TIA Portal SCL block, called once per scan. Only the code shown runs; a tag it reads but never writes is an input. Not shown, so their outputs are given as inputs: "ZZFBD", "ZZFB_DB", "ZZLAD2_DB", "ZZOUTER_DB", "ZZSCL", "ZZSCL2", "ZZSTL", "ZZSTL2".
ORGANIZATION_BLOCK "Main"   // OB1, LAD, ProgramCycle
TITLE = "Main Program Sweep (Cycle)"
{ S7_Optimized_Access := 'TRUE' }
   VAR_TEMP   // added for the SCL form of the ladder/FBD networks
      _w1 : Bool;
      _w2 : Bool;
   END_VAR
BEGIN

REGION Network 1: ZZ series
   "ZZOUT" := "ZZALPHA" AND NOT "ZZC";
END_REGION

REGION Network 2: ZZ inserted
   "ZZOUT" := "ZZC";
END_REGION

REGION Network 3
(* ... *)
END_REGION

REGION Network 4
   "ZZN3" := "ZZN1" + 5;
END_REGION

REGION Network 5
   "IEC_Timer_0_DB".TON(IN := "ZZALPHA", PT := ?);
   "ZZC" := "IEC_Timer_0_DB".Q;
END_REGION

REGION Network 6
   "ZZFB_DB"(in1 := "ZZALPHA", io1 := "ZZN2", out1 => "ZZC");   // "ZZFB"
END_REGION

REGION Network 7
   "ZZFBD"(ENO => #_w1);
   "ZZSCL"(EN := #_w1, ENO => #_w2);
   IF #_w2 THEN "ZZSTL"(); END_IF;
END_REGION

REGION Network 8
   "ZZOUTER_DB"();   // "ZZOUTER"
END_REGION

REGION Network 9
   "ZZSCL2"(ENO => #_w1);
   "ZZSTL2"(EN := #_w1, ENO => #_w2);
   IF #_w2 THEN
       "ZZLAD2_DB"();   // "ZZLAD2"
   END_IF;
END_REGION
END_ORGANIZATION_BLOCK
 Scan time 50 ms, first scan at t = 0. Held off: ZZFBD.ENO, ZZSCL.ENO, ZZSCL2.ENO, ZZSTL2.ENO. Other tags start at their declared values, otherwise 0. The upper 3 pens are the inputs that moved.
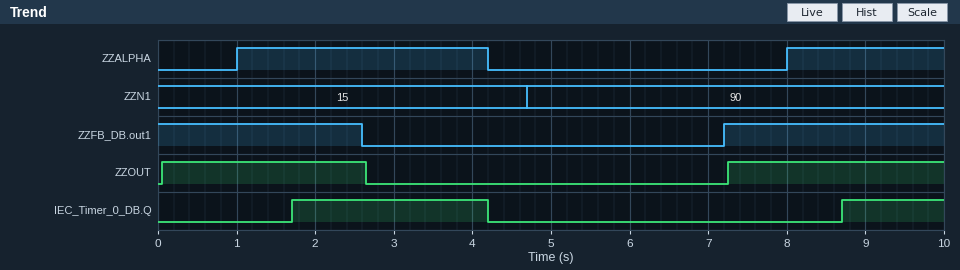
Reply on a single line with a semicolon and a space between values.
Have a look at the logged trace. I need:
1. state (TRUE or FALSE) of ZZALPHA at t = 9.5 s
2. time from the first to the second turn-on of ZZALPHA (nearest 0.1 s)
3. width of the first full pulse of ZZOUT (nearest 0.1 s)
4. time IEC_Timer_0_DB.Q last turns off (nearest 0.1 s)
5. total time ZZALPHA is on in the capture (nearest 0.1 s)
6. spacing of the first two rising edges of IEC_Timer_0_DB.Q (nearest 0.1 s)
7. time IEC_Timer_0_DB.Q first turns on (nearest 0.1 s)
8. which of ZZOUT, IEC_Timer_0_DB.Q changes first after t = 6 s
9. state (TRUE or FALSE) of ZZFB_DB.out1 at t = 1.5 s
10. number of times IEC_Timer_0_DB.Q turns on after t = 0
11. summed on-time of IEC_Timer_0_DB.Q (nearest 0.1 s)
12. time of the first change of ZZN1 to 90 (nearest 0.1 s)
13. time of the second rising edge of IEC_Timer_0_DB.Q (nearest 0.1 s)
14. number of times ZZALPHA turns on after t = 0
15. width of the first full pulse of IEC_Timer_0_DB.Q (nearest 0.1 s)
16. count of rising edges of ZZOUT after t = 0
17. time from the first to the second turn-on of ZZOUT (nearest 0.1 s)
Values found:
TRUE; 7.0 s; 2.6 s; 4.2 s; 5.2 s; 7.0 s; 1.7 s; ZZOUT; TRUE; 2; 3.8 s; 4.7 s; 8.7 s; 2; 2.5 s; 2; 7.2 s
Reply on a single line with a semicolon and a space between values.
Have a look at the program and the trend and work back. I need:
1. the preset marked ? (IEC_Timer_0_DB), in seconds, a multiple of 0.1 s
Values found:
0.7 s
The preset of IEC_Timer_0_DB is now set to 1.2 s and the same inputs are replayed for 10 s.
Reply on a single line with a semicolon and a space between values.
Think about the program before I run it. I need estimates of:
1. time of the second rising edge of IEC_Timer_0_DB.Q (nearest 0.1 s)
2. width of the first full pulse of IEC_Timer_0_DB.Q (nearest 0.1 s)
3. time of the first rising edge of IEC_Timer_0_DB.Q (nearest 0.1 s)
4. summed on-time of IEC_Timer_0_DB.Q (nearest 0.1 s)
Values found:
9.2 s; 2.0 s; 2.2 s; 2.8 s
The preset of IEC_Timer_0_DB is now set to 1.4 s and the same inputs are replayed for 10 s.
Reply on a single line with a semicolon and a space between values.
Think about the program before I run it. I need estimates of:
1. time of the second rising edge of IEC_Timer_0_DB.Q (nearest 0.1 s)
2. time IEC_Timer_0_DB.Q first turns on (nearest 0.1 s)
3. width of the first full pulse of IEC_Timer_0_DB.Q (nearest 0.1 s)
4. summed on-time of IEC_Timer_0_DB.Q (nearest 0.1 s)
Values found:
9.4 s; 2.4 s; 1.8 s; 2.4 s
